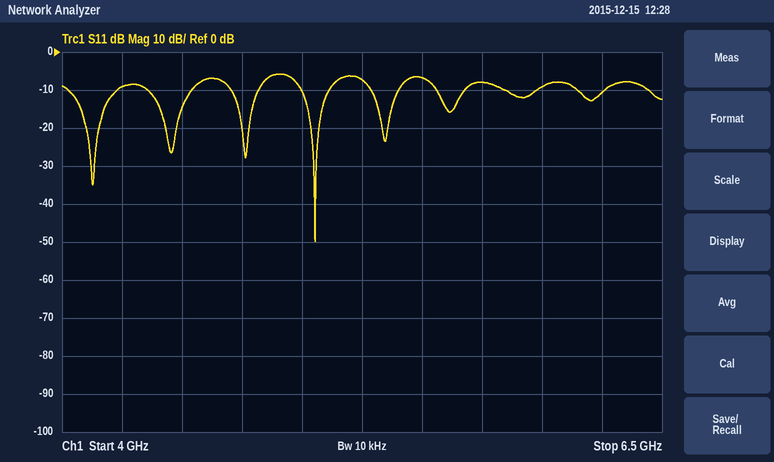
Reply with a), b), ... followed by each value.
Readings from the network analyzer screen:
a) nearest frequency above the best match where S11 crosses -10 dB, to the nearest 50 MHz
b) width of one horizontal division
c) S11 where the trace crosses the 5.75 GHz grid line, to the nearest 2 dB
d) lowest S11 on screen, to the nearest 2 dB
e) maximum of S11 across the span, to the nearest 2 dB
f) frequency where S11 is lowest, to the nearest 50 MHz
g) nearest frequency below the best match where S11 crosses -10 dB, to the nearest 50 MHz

a) 5.10 GHz
b) 250 MHz
c) -8 dB
d) -50 dB
e) -6 dB
f) 5.05 GHz
g) 5.00 GHz
